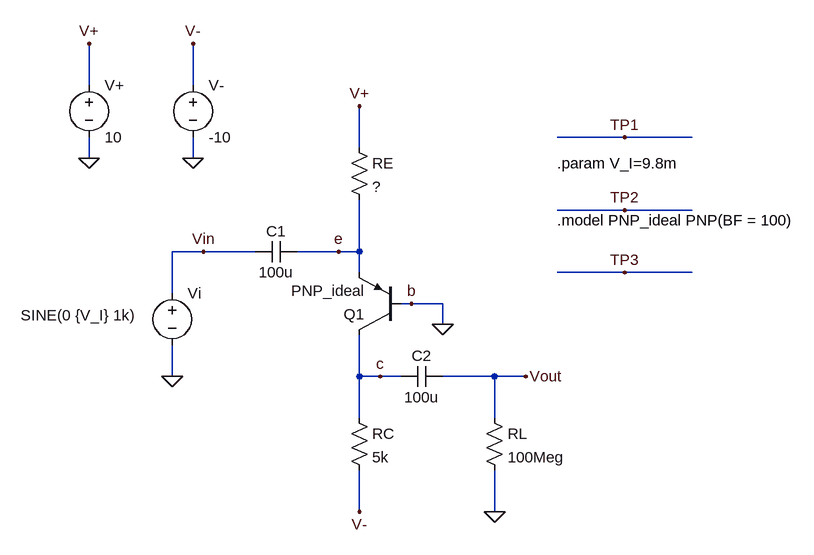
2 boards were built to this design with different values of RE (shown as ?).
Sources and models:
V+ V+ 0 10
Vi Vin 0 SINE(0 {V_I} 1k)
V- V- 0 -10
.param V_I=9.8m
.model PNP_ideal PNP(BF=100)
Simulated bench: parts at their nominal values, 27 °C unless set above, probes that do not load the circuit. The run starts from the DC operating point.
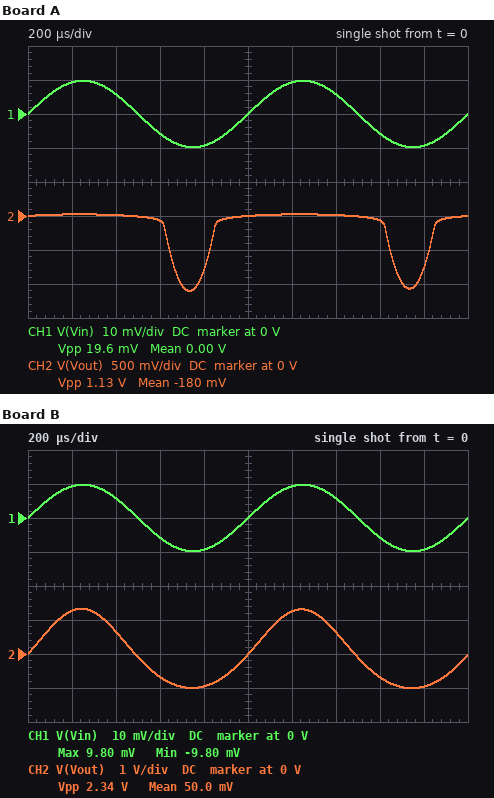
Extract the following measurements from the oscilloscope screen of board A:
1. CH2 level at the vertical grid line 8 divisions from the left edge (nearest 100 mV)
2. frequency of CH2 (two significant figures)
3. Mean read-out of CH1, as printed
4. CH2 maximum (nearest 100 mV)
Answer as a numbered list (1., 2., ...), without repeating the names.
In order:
1. -100 mV
2. 1.0 kHz
3. 0.00 V
4. 0 V
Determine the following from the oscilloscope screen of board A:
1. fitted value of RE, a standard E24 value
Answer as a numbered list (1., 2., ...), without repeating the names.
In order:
1. 3.6 kΩ
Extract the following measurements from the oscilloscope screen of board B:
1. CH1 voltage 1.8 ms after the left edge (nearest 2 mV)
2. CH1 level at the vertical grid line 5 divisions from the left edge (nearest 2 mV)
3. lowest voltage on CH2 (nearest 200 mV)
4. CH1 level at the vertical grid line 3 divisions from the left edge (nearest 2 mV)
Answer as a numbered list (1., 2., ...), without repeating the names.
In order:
1. -10 mV
2. 0 V
3. -1.0 V
4. -6 mV
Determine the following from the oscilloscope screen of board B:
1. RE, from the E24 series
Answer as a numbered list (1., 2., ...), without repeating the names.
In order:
1. 15 kΩ
